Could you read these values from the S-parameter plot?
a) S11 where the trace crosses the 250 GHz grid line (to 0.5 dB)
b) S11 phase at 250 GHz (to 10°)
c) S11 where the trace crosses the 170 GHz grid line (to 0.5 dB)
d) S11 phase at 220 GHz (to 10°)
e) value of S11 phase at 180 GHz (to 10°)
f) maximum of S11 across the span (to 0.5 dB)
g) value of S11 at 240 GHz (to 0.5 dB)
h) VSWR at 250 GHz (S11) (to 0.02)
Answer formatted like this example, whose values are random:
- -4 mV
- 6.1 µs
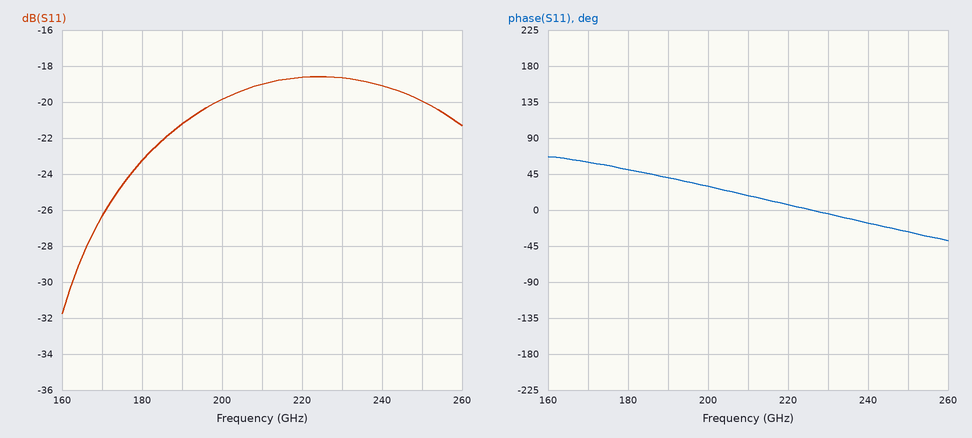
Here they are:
- -20.0 dB
- -30°
- -26.5 dB
- 10°
- 50°
- -18.5 dB
- -19.0 dB
- 1.22
